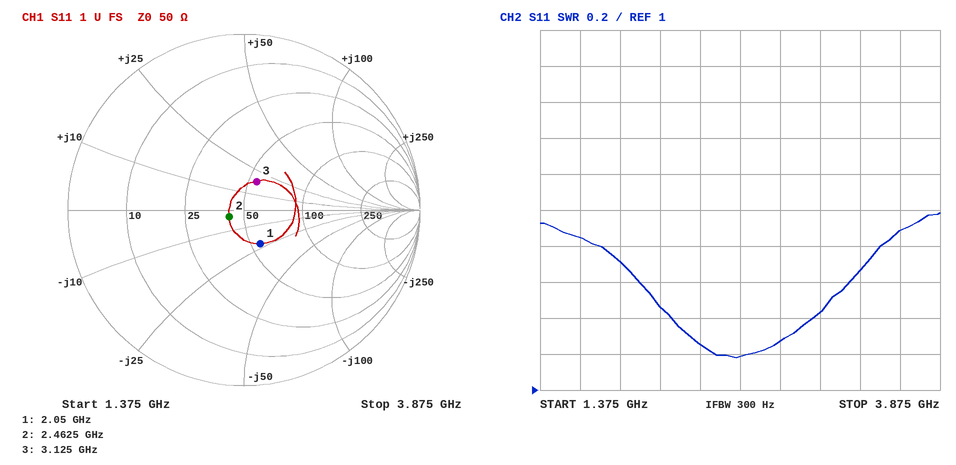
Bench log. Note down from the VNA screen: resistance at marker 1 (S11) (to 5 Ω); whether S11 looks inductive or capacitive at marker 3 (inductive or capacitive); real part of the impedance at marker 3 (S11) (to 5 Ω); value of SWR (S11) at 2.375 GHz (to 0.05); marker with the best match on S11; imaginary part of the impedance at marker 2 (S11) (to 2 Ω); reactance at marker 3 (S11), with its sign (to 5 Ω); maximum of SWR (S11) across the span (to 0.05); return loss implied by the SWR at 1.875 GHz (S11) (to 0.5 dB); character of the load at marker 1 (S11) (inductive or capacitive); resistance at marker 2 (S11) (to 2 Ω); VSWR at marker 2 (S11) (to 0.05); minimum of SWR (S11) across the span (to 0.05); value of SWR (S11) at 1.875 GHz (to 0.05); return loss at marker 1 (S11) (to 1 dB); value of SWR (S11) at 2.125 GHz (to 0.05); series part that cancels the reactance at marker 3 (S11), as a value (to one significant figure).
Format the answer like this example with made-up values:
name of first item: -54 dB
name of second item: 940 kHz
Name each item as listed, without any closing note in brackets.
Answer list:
resistance at marker 1 (S11): 55 Ω
whether S11 looks inductive or capacitive at marker 3: inductive
real part of the impedance at marker 3 (S11): 55 Ω
value of SWR (S11) at 2.375 GHz: 1.25
marker with the best match on S11: marker 2
imaginary part of the impedance at marker 2 (S11): -4 Ω
reactance at marker 3 (S11), with its sign: +20 Ω
maximum of SWR (S11) across the span: 2.00
return loss implied by the SWR at 1.875 GHz (S11): 11.5 dB
character of the load at marker 1 (S11): capacitive
resistance at marker 2 (S11): 42 Ω
VSWR at marker 2 (S11): 1.20
minimum of SWR (S11) across the span: 1.20
value of SWR (S11) at 1.875 GHz: 1.70
return loss at marker 1 (S11): 13 dB
value of SWR (S11) at 2.125 GHz: 1.45
series part that cancels the reactance at marker 3 (S11), as a value: 3 pF
